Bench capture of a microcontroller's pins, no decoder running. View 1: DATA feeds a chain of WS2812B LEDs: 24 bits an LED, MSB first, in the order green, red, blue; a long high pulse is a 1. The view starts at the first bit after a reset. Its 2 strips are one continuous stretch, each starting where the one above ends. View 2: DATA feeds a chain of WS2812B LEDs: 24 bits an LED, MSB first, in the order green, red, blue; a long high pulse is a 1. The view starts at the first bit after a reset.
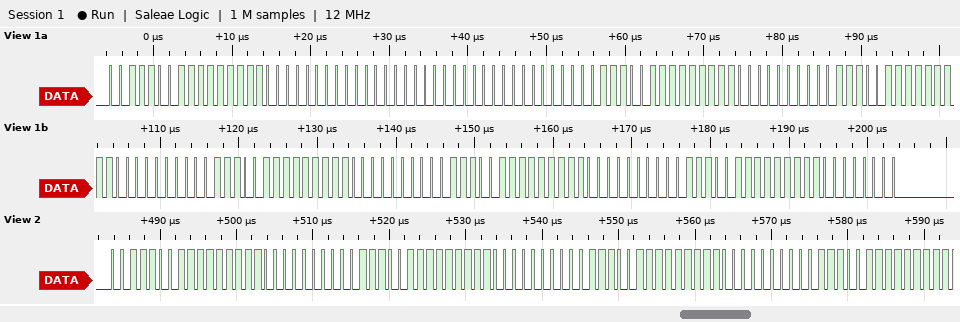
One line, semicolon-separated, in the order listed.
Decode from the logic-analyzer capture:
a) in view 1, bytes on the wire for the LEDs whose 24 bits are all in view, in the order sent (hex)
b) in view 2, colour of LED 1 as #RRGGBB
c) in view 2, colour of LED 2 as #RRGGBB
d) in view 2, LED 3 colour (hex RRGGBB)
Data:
39 FF 00 00 00 00 39 FF 00 39 FF 00 39 FF 00 39 FF 00 39 FF 00; #FF3900; #FF3900; #FF3900
